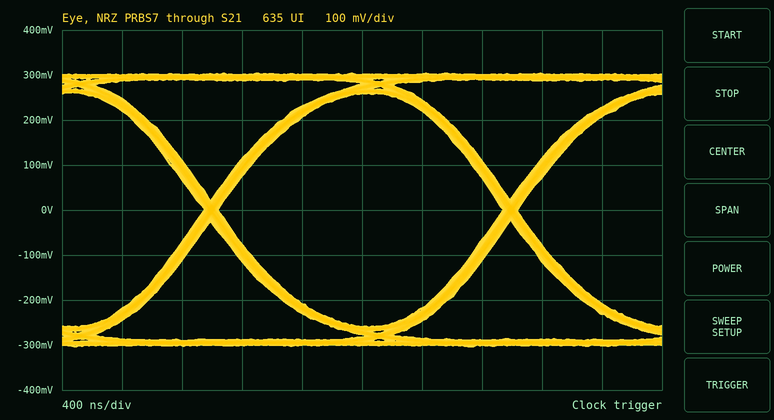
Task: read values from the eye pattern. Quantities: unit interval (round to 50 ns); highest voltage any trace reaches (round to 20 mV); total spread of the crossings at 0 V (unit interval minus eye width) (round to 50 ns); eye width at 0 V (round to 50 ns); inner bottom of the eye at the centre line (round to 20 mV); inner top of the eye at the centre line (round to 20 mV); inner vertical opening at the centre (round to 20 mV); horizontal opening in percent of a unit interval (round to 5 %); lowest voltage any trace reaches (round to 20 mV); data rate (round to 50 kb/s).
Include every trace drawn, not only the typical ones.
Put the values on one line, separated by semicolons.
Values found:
2.00 µs; 300 mV; 100 ns; 1.90 µs; -260 mV; 260 mV; 520 mV; 95 %; -300 mV; 500 kb/s
